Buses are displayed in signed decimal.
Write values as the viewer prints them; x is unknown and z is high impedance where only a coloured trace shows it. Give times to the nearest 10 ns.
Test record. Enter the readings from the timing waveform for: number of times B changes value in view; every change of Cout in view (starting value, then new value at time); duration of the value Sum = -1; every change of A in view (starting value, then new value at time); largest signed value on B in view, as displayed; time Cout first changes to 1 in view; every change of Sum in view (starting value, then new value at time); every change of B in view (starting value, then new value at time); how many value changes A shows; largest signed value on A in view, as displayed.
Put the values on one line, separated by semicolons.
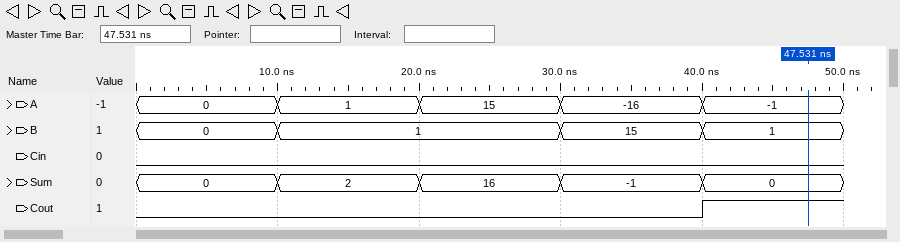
3; 0, 1 at 40 ns; 10 ns; 0, 1 at 10 ns, 15 at 20 ns, -16 at 30 ns, -1 at 40 ns; 15; 40 ns; 0, 2 at 10 ns, 16 at 20 ns, -1 at 30 ns, 0 at 40 ns; 0, 1 at 10 ns, 15 at 30 ns, 1 at 40 ns; 4; 15
